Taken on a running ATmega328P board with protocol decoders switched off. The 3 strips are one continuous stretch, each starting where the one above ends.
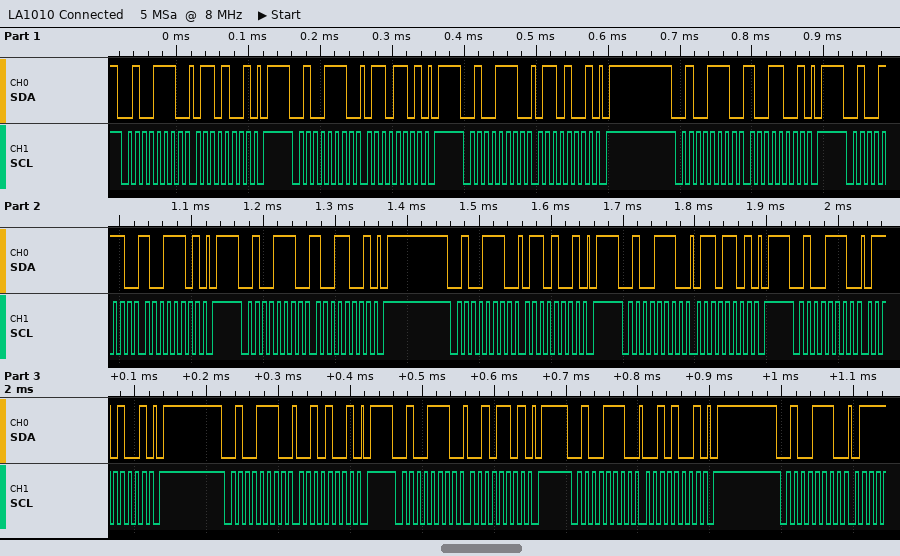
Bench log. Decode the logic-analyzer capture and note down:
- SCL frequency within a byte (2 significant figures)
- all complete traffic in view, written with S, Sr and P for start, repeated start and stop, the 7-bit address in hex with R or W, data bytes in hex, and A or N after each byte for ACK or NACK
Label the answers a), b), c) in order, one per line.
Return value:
a) 100 kHz
b) S 27W A 69 A P S 27W A 6D A P S 27W A 69 A P S 27W A 99 A P S 27W A 9D A P S 27W A 99 A P S 27W A 69 A P S 27W A 6D A P S 27W A 69 A P S 27W A 29 A P S 27W A 2D A P S 27W A 29 A P S 27W A
